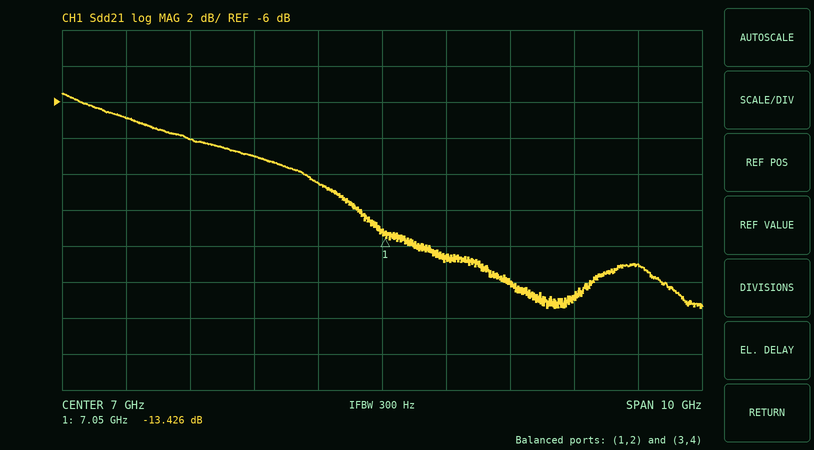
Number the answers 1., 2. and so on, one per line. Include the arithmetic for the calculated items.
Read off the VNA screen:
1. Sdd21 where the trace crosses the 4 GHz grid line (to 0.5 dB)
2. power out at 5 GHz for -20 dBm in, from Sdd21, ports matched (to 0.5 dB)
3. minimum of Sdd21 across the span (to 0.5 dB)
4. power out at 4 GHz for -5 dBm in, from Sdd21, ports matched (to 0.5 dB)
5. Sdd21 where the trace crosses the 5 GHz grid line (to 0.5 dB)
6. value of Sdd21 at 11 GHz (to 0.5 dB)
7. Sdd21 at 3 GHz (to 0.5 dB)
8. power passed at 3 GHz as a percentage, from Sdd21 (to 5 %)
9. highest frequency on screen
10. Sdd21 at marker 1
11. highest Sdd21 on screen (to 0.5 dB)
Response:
1. -8.0 dB
2. -20 dBm + (-9.0 dB) = -29.0 dBm
3. -17.5 dB
4. -5 dBm + (-8.0 dB) = -13.0 dBm
5. -9.0 dB
6. -15.0 dB
7. -7.0 dB
8. 10^(-7/10) ≈ 20 %
9. 12 GHz
10. -13.426 dB
11. -5.5 dB
